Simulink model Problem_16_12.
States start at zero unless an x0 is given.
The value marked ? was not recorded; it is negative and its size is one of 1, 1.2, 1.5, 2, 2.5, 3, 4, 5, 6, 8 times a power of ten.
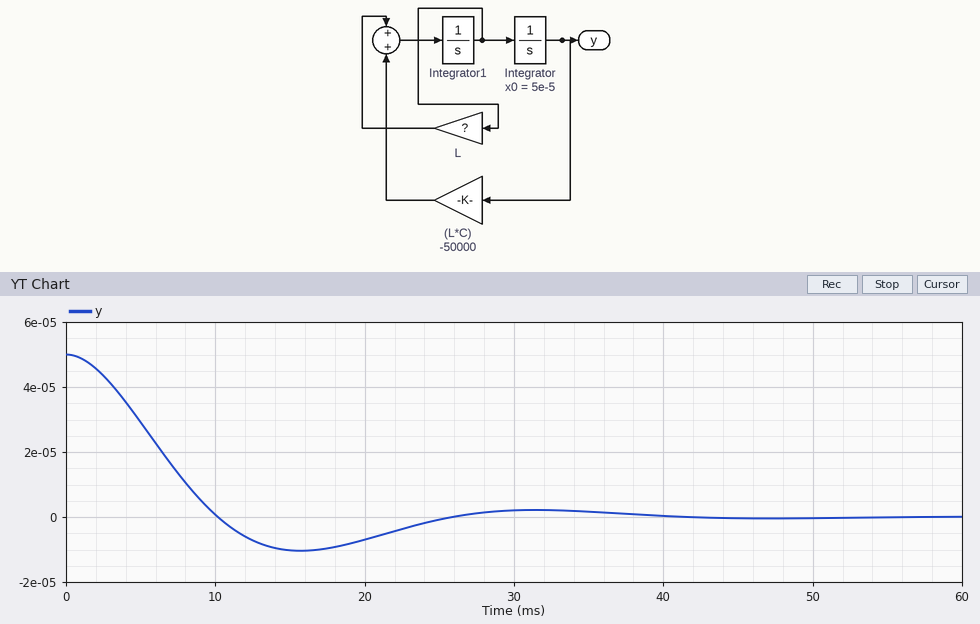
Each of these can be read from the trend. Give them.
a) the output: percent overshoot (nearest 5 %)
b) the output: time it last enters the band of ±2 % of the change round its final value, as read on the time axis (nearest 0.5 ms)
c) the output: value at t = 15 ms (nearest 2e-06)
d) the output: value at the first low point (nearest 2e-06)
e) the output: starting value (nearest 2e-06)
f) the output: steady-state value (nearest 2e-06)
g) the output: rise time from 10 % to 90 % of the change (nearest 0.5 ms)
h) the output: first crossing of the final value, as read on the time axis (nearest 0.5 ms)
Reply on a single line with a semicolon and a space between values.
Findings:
20 %; 37.5 ms; -0.000010; -0.000010; 0.000050; 0.000000; 7.0 ms; 10.0 ms
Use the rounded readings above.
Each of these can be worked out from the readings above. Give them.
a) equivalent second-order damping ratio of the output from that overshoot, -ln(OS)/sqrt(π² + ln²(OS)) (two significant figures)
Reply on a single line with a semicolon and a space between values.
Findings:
0.46
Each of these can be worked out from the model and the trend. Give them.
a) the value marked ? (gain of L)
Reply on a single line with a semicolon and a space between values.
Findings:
-200
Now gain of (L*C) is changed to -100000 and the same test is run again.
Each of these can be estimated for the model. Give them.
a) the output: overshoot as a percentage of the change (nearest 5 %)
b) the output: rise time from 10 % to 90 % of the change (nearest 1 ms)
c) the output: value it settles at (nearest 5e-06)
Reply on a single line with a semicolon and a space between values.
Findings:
35 %; 4 ms; 0.000000
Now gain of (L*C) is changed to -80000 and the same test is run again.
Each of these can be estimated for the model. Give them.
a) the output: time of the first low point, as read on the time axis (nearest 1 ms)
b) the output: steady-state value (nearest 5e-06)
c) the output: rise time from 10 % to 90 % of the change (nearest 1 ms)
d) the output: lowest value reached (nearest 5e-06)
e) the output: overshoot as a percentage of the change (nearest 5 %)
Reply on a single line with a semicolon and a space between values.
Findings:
12 ms; 0.000000; 5 ms; -0.000015; 30 %
